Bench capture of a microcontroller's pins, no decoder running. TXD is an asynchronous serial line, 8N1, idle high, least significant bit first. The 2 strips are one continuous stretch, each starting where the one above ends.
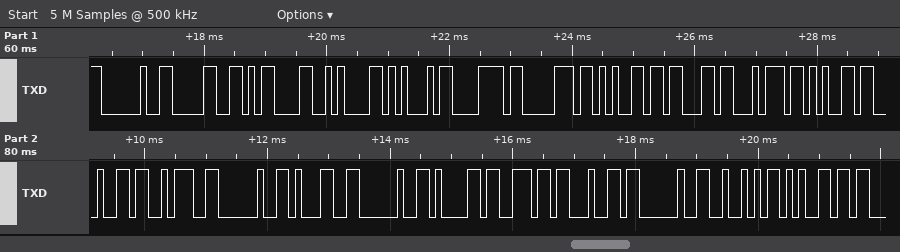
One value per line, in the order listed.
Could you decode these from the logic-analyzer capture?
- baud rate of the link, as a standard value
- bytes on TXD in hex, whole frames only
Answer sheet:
9600 baud
0x20 0x30 0x0D 0x0A 0x45 0x78 0x70 0x65 0x63 0x74 0x65 0x64 0x3A 0x20 0x31 0x20 0x61 0x6E 0x64 0x20 0x52 0x65
